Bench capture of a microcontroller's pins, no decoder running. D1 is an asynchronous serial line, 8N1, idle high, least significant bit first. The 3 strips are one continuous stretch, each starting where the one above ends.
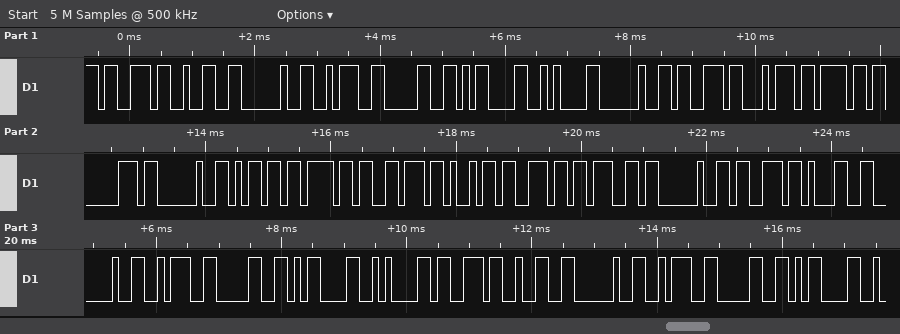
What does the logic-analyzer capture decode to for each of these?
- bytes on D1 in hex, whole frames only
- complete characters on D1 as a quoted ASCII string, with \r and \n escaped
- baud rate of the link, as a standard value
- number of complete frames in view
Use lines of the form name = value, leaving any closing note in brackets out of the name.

bytes on D1 in hex, whole frames only = 0x73 0x32 0x20 0x3A 0x30 0x0D 0x0A 0x20 0x73 0x74 0x6F 0x70 0x20 0x6D 0x6F 0x76 0x69 0x6E 0x67 0x20 0x73 0x31 0x20 0x3A 0x30 0x0D 0x0A 0x73 0x32 0x20 0x3A 0x30 0x0D
complete characters on D1 as a quoted ASCII string, with \r and \n escaped = "s2 :0\r\n stop moving s1 :0\r\ns2 :0\r"
baud rate of the link, as a standard value = 9600 baud
number of complete frames in view = 33
